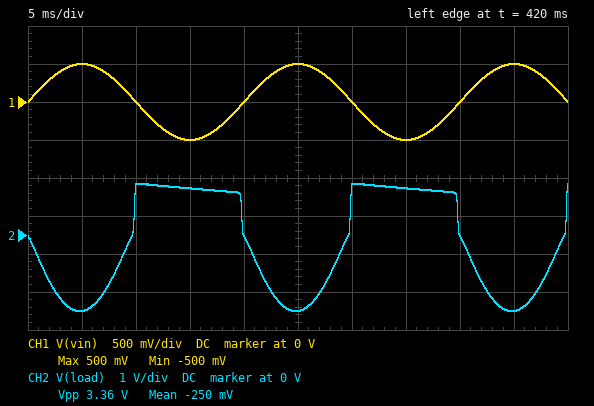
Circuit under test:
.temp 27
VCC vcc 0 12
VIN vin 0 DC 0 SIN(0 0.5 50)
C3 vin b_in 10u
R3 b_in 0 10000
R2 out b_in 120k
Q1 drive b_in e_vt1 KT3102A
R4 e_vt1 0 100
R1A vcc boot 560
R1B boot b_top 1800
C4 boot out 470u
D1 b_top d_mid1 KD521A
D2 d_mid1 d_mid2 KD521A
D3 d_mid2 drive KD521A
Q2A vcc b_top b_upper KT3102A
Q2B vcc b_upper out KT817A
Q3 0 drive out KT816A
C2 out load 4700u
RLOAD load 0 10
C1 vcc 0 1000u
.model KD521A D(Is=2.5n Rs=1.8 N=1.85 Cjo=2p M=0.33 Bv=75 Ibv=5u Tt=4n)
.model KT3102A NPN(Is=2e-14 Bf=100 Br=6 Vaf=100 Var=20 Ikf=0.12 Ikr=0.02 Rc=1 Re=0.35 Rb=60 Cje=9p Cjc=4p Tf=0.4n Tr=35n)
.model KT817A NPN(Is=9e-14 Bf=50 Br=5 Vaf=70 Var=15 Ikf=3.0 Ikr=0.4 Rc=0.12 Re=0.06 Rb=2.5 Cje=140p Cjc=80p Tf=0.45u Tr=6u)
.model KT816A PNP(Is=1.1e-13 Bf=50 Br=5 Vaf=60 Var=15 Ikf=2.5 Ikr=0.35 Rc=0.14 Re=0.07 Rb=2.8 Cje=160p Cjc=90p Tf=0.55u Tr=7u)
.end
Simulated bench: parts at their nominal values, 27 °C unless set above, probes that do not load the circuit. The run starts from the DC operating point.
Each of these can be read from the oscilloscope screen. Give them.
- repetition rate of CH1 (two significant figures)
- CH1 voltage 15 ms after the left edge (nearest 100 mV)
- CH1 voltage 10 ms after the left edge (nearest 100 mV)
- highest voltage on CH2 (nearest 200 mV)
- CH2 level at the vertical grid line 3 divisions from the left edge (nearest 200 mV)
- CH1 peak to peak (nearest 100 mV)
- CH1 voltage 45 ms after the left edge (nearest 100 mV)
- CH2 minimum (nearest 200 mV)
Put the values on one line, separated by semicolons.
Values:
50 Hz; -500 mV; 0 V; 1.4 V; 1.2 V; 1.0 V; 500 mV; -2.0 V
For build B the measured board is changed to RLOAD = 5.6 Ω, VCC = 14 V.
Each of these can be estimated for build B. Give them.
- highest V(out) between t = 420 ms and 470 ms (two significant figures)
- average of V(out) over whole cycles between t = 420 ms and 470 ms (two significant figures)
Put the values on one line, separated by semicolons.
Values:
13 V; 12 V
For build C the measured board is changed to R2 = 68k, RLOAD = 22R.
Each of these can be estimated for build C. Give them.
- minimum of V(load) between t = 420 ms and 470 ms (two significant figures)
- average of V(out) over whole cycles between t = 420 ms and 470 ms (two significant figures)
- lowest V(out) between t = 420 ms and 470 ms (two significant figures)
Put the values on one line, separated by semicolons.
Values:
-4.7 V; 7.9 V; 3.2 V
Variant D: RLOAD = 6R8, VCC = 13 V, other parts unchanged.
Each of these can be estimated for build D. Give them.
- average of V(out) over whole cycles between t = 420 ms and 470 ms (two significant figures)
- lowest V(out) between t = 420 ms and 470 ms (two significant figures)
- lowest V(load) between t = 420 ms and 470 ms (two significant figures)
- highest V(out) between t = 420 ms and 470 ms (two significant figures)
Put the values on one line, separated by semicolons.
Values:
11 V; 9.5 V; -1.6 V; 12 V
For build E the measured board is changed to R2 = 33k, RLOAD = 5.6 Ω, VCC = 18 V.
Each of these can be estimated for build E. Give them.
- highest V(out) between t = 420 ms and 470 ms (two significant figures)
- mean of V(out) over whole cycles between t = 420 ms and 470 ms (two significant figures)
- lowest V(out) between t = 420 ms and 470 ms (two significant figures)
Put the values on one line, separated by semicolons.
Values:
16 V; 8.7 V; 6.5 V
